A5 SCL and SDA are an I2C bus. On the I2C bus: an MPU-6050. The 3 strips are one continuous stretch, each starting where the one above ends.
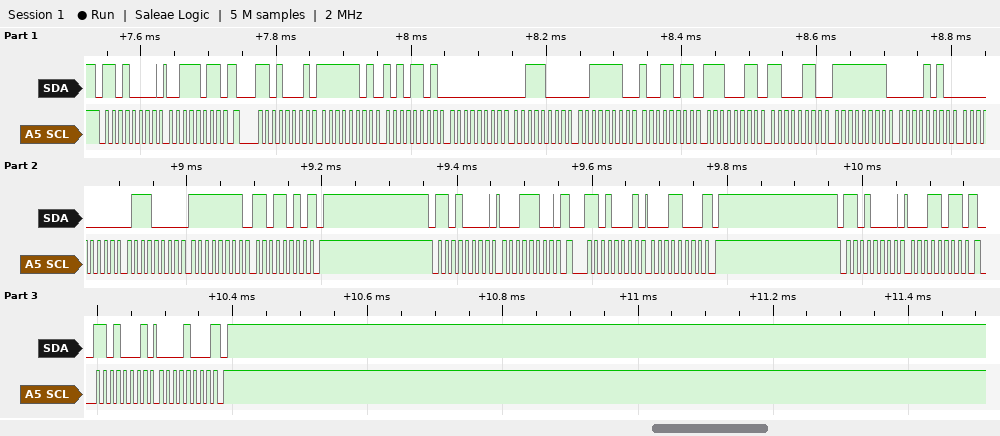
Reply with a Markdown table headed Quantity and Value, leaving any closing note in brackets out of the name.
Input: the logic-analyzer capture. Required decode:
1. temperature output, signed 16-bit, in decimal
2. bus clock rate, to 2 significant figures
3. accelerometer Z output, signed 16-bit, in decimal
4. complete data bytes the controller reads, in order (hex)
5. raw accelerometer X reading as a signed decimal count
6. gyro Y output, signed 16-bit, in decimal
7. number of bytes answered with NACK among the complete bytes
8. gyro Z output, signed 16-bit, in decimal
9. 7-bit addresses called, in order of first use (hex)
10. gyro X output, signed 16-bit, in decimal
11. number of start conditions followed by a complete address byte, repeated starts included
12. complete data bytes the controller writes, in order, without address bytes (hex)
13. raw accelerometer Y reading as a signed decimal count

| Quantity | Value |
|---|---|
| temperature output, signed 16-bit, in decimal | -7226 |
| bus clock rate, to 2 significant figures | 100 kHz |
| accelerometer Z output, signed 16-bit, in decimal | 16027 |
| complete data bytes the controller reads, in order | FD AD 00 38 3E 9B E3 C6 FF 0A 00 70 FF DA 18 08 |
| raw accelerometer X reading as a signed decimal count | -595 |
| gyro Y output, signed 16-bit, in decimal | 112 |
| number of bytes answered with NACK among the complete bytes | 3 |
| gyro Z output, signed 16-bit, in decimal | -38 |
| 7-bit addresses called, in order of first use | 0x68 |
| gyro X output, signed 16-bit, in decimal | -246 |
| number of start conditions followed by a complete address byte, repeated starts included | 6 |
| complete data bytes the controller writes, in order, without address bytes | 3B 1C 1B |
| raw accelerometer Y reading as a signed decimal count | 56 |
